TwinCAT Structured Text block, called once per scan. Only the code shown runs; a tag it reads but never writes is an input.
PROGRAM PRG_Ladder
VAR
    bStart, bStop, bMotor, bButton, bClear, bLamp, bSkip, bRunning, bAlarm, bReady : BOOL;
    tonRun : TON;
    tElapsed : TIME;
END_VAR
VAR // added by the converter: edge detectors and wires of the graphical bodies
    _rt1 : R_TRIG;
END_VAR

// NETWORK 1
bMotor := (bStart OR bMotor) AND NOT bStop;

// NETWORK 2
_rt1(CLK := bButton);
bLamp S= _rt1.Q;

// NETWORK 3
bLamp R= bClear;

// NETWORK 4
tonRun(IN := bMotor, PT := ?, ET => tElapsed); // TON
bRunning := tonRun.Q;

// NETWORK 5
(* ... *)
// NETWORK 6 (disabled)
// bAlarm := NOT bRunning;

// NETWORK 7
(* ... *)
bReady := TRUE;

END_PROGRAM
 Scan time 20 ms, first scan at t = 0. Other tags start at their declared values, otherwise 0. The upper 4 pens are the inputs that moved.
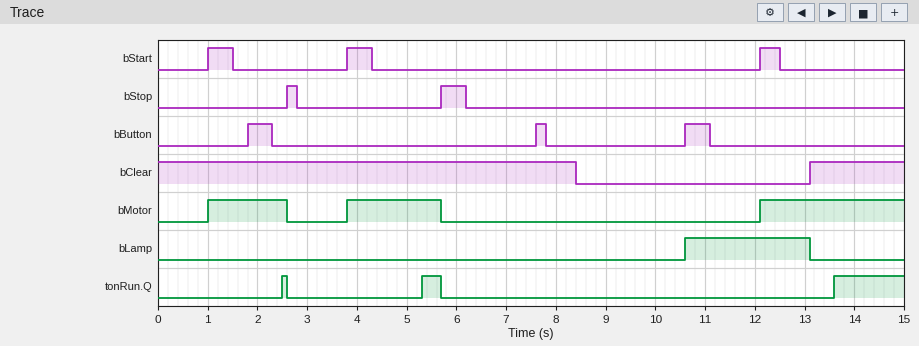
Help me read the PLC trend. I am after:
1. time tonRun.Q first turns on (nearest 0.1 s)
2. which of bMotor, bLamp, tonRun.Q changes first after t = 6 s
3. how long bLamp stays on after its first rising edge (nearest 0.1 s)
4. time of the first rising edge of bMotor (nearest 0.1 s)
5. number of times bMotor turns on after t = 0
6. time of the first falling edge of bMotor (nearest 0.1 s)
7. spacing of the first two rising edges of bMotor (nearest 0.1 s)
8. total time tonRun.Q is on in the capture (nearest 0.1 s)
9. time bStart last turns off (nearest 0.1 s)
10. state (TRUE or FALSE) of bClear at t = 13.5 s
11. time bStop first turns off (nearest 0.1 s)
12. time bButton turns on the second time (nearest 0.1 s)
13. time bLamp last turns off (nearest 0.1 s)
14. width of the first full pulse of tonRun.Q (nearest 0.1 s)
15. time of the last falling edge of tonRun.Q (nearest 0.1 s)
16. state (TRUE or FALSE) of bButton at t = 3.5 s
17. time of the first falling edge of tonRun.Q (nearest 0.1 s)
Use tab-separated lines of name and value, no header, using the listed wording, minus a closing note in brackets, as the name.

time tonRun.Q first turns on	2.5 s
which of bMotor, bLamp, tonRun.Q changes first after t = 6 s	bLamp
how long bLamp stays on after its first rising edge	2.5 s
time of the first rising edge of bMotor	1.0 s
number of times bMotor turns on after t = 0	3
time of the first falling edge of bMotor	2.6 s
spacing of the first two rising edges of bMotor	2.8 s
total time tonRun.Q is on in the capture	1.9 s
time bStart last turns off	12.5 s
state (TRUE or FALSE) of bClear at t = 13.5 s	TRUE
time bStop first turns off	2.8 s
time bButton turns on the second time	7.6 s
time bLamp last turns off	13.1 s
width of the first full pulse of tonRun.Q	0.1 s
time of the last falling edge of tonRun.Q	5.7 s
state (TRUE or FALSE) of bButton at t = 3.5 s	FALSE
time of the first falling edge of tonRun.Q	2.6 s
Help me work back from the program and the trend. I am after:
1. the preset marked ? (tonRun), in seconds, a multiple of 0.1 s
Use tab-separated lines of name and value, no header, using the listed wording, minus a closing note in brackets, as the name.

the preset marked ? (tonRun), in seconds, a multiple of 0.1 s	1.5 s
